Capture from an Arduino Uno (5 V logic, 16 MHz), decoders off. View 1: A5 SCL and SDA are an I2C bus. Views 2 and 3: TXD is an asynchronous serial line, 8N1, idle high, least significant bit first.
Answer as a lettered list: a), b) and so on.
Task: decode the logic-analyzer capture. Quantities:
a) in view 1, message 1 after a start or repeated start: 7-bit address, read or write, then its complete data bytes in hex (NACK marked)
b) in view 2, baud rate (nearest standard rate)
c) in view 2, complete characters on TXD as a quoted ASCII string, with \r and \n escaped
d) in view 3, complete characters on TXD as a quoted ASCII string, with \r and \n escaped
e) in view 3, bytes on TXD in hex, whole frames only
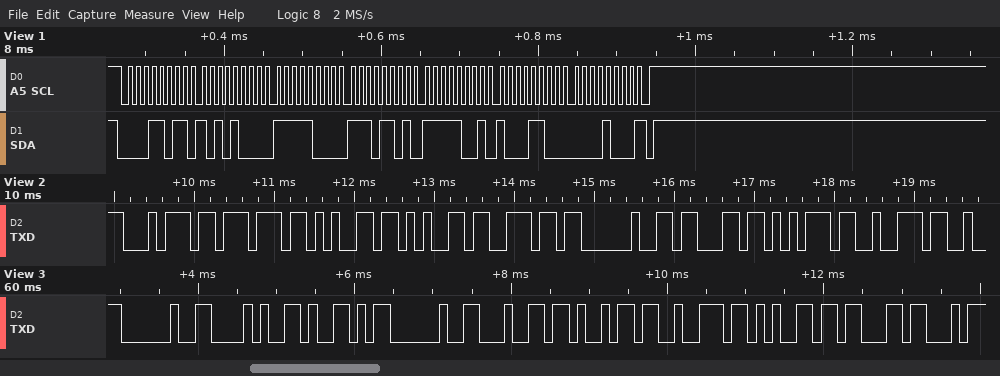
a) 0x0D read: A8 F8 ED F9 8C 08 NACK
b) 9600 baud
c) "tween cur"
d) " (Y direc"
e) 20 28 59 20 64 69 72 65 63
